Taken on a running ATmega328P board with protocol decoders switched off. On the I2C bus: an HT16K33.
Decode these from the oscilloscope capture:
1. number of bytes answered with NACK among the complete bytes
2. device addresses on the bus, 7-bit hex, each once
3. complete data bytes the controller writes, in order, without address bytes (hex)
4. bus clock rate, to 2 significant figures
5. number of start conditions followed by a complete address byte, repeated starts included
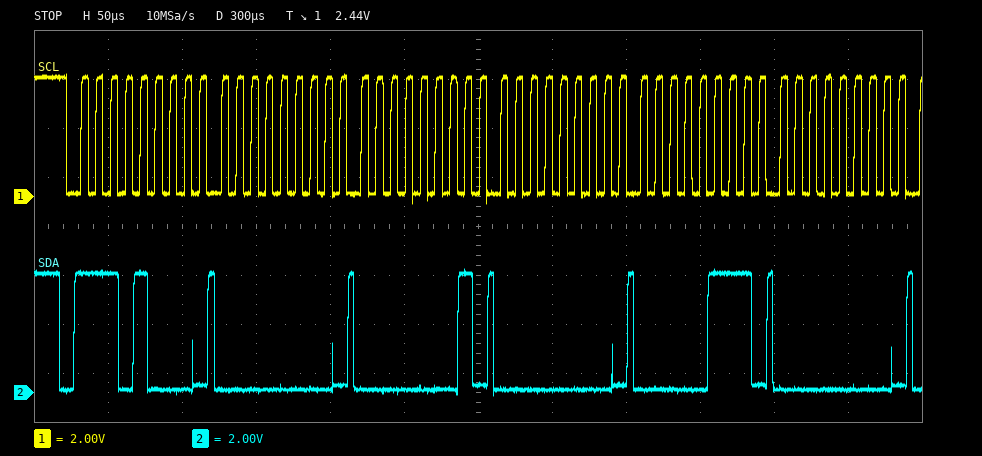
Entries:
0
0x74
00 01 00 07 00
100 kHz
1
